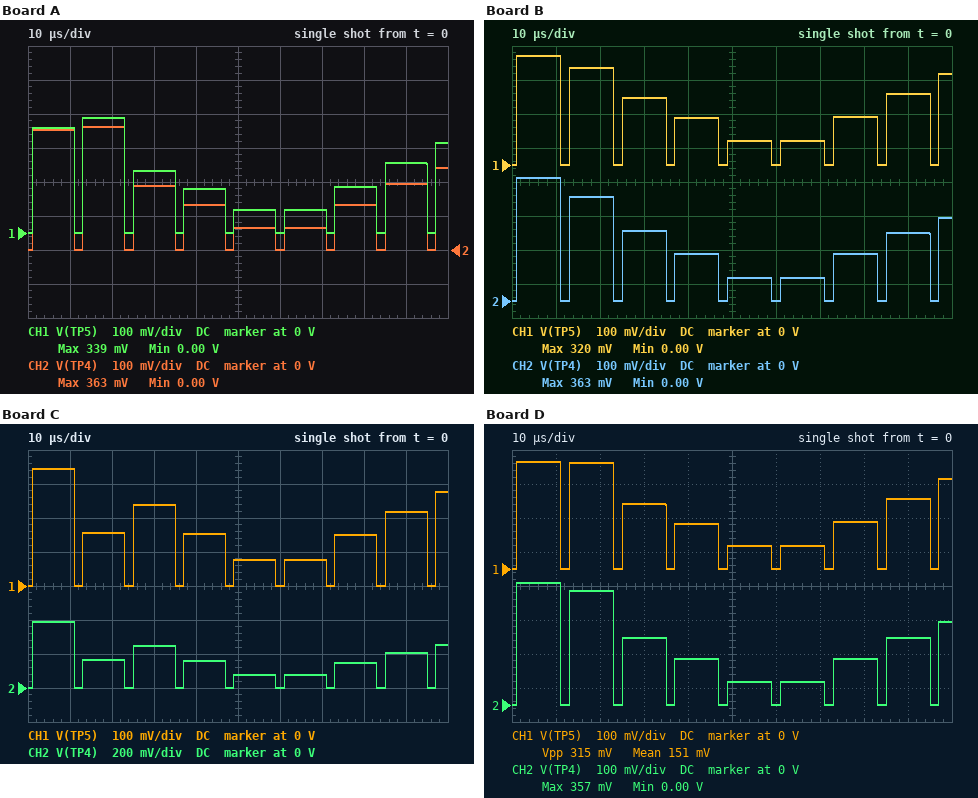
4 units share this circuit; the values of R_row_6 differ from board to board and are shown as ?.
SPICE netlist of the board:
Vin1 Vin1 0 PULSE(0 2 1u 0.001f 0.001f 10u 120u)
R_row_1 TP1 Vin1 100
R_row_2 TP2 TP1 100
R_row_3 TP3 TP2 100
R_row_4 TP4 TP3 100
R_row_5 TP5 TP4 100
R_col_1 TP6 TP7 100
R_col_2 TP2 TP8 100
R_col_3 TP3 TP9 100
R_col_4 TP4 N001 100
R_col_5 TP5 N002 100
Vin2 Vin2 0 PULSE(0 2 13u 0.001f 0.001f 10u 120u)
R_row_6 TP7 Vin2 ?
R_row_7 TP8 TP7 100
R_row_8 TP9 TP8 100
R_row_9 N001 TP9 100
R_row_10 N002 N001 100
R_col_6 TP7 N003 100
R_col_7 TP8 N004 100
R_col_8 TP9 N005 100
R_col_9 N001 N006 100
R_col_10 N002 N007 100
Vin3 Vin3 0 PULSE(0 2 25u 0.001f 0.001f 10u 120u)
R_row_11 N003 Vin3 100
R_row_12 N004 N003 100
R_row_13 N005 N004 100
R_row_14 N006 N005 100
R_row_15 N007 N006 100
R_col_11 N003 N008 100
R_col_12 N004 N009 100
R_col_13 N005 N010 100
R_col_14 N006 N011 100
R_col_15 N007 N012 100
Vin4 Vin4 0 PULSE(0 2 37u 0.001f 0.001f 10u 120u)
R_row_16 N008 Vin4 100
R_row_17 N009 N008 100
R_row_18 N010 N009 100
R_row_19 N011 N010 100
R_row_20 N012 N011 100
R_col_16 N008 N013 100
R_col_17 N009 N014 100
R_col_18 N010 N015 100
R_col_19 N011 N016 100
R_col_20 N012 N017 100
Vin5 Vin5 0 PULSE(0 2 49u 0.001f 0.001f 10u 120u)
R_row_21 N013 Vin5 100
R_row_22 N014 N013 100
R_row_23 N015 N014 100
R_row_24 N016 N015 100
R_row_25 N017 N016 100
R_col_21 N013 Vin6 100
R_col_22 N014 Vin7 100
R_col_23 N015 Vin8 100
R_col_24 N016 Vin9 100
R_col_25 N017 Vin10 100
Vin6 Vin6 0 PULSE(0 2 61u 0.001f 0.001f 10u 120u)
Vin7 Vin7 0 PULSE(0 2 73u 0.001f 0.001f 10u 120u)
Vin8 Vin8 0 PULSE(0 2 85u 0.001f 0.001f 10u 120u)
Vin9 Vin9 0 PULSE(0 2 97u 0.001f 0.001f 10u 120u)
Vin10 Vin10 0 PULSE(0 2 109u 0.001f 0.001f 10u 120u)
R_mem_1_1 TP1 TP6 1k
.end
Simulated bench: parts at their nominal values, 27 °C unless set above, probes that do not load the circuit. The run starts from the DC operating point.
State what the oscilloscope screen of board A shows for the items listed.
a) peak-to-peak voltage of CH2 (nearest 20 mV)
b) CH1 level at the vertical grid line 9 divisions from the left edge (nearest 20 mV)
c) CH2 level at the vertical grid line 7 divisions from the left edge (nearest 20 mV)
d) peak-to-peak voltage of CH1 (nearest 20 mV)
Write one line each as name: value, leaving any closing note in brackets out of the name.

peak-to-peak voltage of CH2: 360 mV
CH1 level at the vertical grid line 9 divisions from the left edge: 200 mV
CH2 level at the vertical grid line 7 divisions from the left edge: 60 mV
peak-to-peak voltage of CH1: 340 mV
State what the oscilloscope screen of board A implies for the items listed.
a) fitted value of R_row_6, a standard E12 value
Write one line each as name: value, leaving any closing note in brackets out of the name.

fitted value of R_row_6, a standard E12 value: 56 Ω
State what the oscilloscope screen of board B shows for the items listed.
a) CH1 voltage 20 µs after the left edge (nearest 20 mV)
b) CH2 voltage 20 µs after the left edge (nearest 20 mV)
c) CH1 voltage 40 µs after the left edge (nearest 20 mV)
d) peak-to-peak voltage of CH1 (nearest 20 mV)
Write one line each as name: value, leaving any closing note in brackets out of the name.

CH1 voltage 20 µs after the left edge: 280 mV
CH2 voltage 20 µs after the left edge: 300 mV
CH1 voltage 40 µs after the left edge: 140 mV
peak-to-peak voltage of CH1: 320 mV
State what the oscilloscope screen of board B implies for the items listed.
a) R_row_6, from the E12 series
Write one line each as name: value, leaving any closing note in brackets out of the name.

R_row_6, from the E12 series: 82 Ω
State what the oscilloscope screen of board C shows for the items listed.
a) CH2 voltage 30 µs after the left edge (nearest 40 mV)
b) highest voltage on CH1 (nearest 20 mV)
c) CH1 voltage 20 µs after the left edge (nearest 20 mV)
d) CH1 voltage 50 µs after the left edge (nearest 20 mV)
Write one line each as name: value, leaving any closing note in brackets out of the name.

CH2 voltage 30 µs after the left edge: 240 mV
highest voltage on CH1: 340 mV
CH1 voltage 20 µs after the left edge: 160 mV
CH1 voltage 50 µs after the left edge: 80 mV
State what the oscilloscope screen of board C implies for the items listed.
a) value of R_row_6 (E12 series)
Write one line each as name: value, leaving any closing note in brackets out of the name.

value of R_row_6: 220 Ω
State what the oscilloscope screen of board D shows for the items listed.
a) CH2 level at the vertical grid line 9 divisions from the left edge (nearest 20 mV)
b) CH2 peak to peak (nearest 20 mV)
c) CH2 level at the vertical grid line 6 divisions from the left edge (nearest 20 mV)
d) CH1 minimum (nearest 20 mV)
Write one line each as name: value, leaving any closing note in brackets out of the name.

CH2 level at the vertical grid line 9 divisions from the left edge: 200 mV
CH2 peak to peak: 360 mV
CH2 level at the vertical grid line 6 divisions from the left edge: 0 V
CH1 minimum: 0 V
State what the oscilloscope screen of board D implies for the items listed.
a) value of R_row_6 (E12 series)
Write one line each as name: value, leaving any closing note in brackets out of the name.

value of R_row_6: 68 Ω
